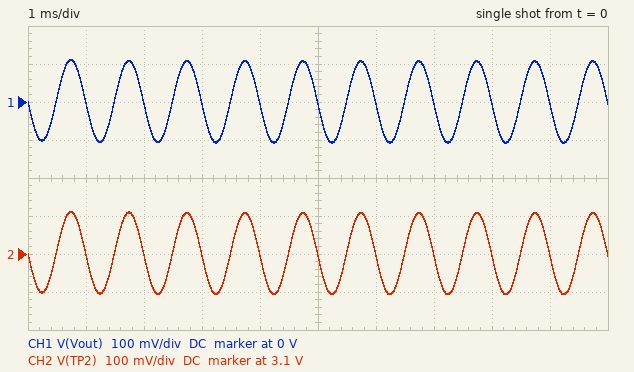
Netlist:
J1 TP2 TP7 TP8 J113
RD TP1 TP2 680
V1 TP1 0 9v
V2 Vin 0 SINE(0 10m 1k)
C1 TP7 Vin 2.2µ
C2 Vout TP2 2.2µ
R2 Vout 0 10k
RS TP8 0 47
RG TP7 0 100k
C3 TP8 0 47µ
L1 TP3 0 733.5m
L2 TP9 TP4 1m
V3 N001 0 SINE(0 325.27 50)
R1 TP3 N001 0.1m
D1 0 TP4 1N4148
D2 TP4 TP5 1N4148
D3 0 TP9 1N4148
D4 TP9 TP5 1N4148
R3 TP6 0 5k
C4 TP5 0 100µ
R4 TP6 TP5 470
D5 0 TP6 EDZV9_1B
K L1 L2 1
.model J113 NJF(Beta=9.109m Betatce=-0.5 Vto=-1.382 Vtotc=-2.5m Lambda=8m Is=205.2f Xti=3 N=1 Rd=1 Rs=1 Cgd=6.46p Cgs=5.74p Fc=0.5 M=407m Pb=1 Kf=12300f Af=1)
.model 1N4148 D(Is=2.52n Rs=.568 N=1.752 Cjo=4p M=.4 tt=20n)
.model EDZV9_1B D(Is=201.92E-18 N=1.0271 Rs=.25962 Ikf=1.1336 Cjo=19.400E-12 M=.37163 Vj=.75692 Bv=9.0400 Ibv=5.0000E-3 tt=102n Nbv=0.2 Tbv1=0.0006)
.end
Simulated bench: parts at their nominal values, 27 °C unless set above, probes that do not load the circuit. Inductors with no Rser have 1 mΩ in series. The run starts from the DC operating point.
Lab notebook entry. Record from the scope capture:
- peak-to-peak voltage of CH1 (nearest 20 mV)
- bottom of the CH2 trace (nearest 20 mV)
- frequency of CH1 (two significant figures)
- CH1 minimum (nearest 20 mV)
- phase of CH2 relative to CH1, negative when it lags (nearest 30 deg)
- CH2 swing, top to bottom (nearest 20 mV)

220 mV
3.00 V
1.0 kHz
-100 mV
0 deg
220 mV
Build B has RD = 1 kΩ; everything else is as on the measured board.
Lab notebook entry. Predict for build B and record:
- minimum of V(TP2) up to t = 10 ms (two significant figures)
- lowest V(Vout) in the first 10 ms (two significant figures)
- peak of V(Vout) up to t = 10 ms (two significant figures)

1.0 V
-15 mV
16 mV
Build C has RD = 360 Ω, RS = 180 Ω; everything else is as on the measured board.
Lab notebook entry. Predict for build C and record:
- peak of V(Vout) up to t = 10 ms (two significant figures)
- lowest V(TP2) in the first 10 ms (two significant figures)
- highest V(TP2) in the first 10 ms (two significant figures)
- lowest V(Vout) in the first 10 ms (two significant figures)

44 mV
7.5 V
7.6 V
-42 mV
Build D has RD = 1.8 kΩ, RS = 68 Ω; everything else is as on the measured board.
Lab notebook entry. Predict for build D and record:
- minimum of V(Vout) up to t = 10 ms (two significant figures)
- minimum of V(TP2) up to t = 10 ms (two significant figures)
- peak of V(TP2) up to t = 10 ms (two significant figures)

-3.3 mV
600 mV
610 mV
